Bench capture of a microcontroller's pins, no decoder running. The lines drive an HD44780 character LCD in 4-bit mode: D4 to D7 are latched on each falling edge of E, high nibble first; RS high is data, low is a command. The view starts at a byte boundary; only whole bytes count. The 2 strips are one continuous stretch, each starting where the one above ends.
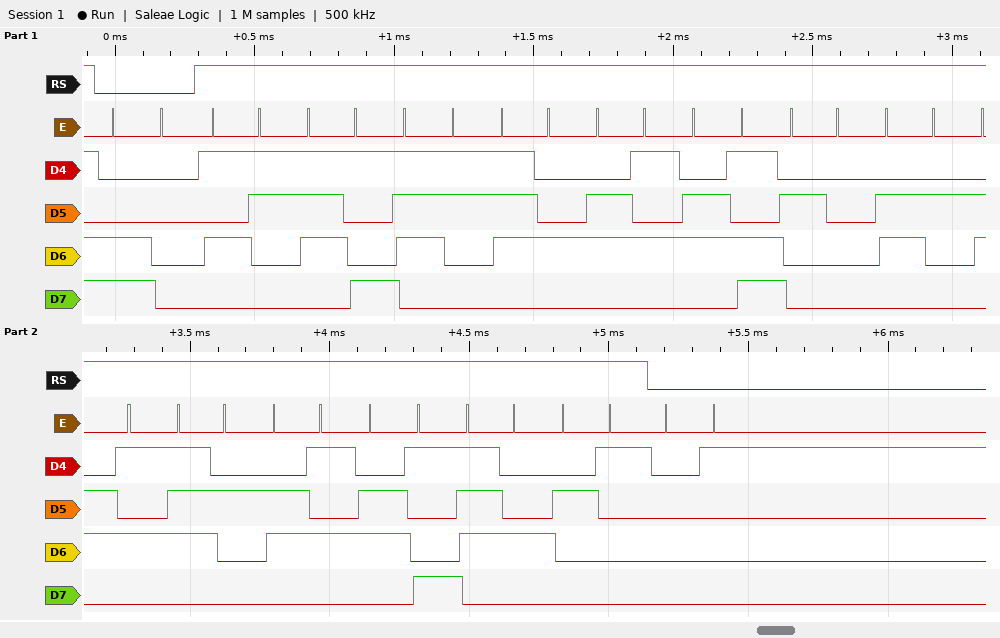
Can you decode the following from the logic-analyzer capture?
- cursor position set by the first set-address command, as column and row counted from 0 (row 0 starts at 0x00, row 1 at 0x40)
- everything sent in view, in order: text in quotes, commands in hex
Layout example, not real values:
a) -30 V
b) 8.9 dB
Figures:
a) column 0, row 1
b) 0xC0 "System bereit!" 0x01
